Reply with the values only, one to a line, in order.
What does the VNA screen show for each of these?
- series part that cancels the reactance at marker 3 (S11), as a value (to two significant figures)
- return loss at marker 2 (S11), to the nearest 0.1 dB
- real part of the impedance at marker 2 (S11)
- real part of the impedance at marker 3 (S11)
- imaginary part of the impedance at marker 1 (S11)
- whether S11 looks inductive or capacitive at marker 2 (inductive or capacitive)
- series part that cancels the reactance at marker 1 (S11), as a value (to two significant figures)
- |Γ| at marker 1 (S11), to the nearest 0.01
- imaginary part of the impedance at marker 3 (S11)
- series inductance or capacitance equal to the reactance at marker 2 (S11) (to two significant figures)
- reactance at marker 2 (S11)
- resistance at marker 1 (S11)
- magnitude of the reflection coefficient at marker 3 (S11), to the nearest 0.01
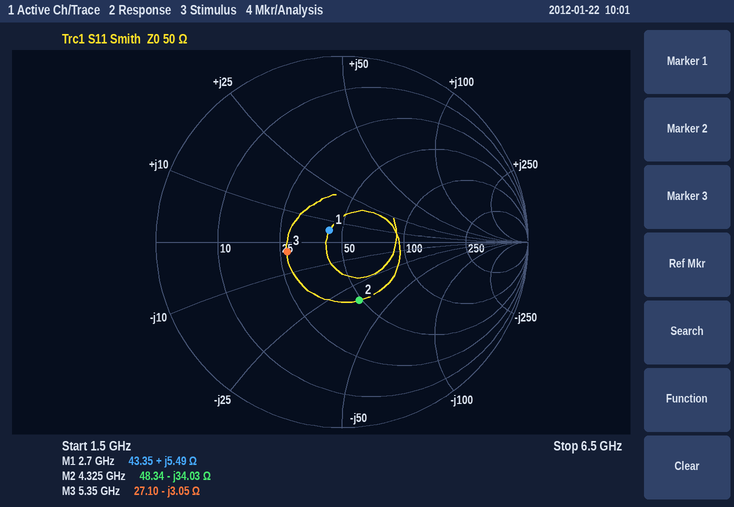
91 pH
9.7 dB
48.34 Ω
27.10 Ω
+5.49 Ω
capacitive
11 pF
0.09
-3.05 Ω
1.1 pF
-34.03 Ω
43.35 Ω
0.30
